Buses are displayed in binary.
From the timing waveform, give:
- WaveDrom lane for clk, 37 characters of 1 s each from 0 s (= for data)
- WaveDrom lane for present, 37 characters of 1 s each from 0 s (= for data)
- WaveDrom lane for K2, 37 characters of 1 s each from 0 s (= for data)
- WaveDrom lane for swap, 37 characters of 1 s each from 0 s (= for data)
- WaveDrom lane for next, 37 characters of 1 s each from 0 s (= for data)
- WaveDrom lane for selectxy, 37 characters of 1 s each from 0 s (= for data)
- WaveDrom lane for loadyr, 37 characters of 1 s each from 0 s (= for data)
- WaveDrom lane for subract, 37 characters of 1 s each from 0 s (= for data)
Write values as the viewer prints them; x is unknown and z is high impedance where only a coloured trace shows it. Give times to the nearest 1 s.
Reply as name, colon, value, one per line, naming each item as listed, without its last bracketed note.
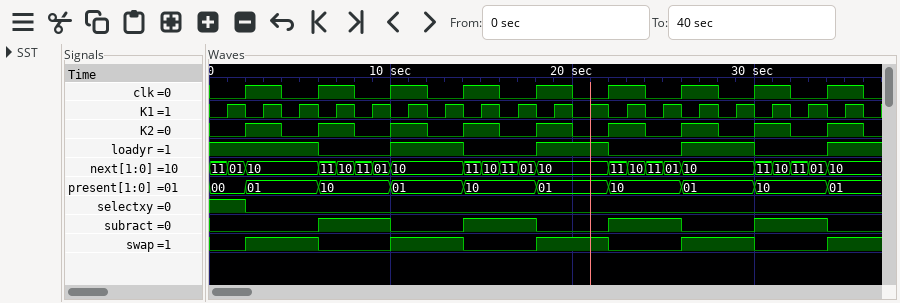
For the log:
WaveDrom lane for clk, 37 characters of 1 s each from 0 s: {name: 'clk', wave: '0.1.0.1.0.1.0.1.0.1.0.1.0.1.0.1.0.1.0'}
WaveDrom lane for present, 37 characters of 1 s each from 0 s: {name: 'present', wave: '=.=...=...=...=...=...=...=...=...=..', data: '00 01 10 01 10 01 10 01 10 01'}
WaveDrom lane for K2, 37 characters of 1 s each from 0 s: {name: 'K2', wave: '0.1.0.1.0.1.0.1.0.1.0.1.0.1.0.1.0.1.0'}
WaveDrom lane for swap, 37 characters of 1 s each from 0 s: {name: 'swap', wave: '0.1...0...1...0...1...0...1...0...1..'}
WaveDrom lane for next, 37 characters of 1 s each from 0 s: {name: 'next', wave: '===...=====...=====...=====...=====..', data: '11 01 10 11 10 11 01 10 11 10 11 01 10 11 10 11 01 10 11 10 11 01 10'}
WaveDrom lane for selectxy, 37 characters of 1 s each from 0 s: {name: 'selectxy', wave: '1.0..................................'}
WaveDrom lane for loadyr, 37 characters of 1 s each from 0 s: {name: 'loadyr', wave: '1.....0...1...0...1...0...1...0...1..'}
WaveDrom lane for subract, 37 characters of 1 s each from 0 s: {name: 'subract', wave: '0.....1...0...1...0...1...0...1...0..'}
